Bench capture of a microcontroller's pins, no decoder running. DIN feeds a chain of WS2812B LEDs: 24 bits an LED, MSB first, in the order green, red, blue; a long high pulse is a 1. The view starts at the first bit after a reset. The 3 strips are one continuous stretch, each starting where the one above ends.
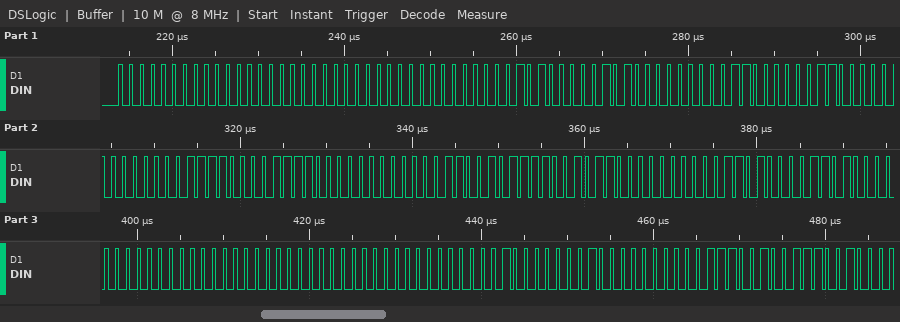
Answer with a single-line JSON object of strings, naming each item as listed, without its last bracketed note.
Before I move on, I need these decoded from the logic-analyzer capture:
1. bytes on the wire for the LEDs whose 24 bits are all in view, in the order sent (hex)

{"bytes on the wire for the LEDs whose 24 bits are all in view, in the order sent": "00 00 00 00 05 05 00 60 60 00 F0 F0 00 CB CB 00 34 34 00 00 00 00 01 01 00 39 39"}
